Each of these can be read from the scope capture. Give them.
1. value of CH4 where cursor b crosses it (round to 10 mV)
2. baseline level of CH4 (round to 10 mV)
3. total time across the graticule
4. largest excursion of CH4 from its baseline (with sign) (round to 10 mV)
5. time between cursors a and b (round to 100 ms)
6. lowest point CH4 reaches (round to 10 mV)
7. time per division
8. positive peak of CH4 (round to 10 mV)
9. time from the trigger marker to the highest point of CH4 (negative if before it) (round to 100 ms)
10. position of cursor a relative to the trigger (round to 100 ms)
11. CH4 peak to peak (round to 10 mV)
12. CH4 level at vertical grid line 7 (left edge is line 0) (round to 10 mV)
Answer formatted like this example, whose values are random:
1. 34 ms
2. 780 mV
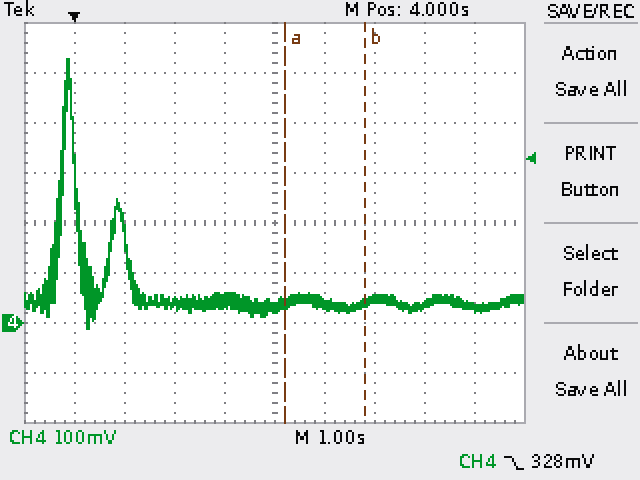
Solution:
1. 40 mV
2. 40 mV
3. 10 s
4. +490 mV
5. 1.6 s
6. -10 mV
7. 1 s
8. 530 mV
9. -100 ms
10. +4.2 s
11. 540 mV
12. 50 mV
